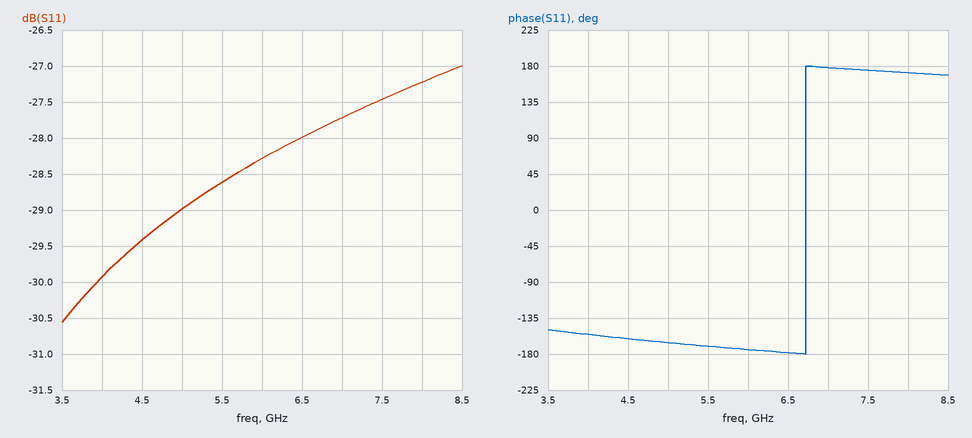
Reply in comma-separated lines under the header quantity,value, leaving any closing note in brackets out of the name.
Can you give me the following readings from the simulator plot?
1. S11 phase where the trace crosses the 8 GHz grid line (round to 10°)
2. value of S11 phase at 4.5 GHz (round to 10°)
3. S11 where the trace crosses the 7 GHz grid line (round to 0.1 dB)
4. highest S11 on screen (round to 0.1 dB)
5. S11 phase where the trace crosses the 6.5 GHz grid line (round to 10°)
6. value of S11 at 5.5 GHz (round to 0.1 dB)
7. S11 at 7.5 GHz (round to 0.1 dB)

quantity,value
S11 phase where the trace crosses the 8 GHz grid line,170°
value of S11 phase at 4.5 GHz,-160°
S11 where the trace crosses the 7 GHz grid line,-27.7 dB
highest S11 on screen,-27.0 dB
S11 phase where the trace crosses the 6.5 GHz grid line,-180°
value of S11 at 5.5 GHz,-28.6 dB
S11 at 7.5 GHz,-27.5 dB
